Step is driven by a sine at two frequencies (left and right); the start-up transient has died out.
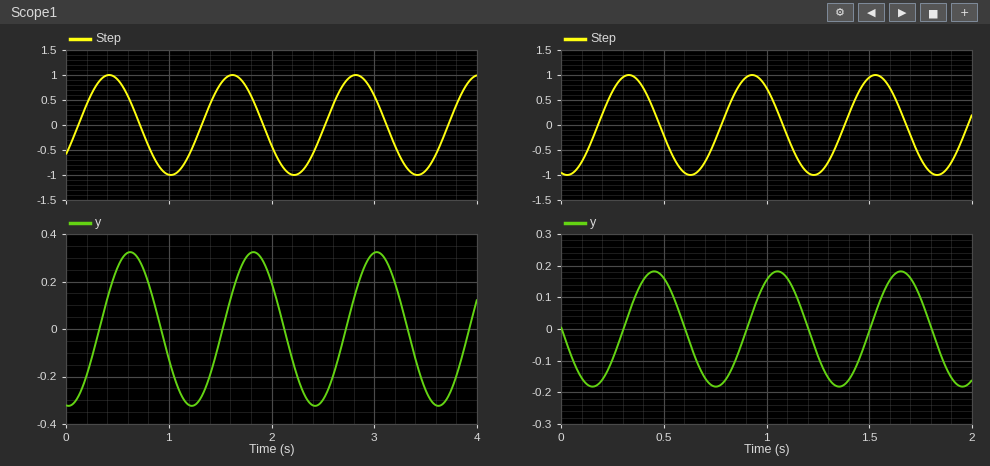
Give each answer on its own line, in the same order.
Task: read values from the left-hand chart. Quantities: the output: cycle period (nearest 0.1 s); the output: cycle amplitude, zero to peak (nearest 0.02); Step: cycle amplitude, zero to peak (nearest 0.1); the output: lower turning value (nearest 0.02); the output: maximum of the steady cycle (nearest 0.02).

1.2 s
0.32
1.0
-0.32
0.32
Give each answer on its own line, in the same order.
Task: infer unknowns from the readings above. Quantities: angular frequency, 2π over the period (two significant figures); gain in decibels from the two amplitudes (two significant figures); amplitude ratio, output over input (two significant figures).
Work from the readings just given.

5.2 rad/s
-9.9 dB
0.32
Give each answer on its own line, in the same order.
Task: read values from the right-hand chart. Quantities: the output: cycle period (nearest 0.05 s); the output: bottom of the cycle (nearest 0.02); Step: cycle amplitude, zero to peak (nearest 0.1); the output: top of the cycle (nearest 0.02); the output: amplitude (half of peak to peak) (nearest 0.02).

0.60 s
-0.18
1.0
0.18
0.18
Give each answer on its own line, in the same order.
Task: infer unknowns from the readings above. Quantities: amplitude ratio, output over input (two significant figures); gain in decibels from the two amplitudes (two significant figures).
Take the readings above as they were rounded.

0.18
-15 dB
